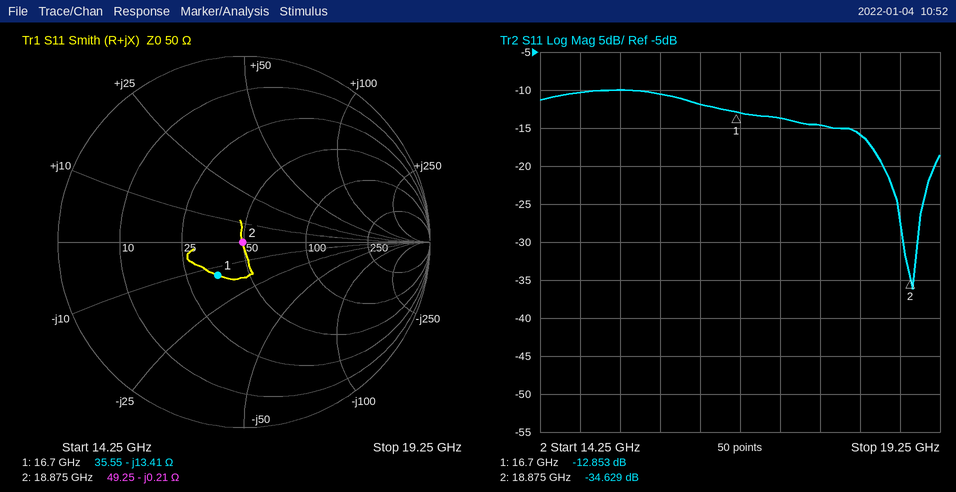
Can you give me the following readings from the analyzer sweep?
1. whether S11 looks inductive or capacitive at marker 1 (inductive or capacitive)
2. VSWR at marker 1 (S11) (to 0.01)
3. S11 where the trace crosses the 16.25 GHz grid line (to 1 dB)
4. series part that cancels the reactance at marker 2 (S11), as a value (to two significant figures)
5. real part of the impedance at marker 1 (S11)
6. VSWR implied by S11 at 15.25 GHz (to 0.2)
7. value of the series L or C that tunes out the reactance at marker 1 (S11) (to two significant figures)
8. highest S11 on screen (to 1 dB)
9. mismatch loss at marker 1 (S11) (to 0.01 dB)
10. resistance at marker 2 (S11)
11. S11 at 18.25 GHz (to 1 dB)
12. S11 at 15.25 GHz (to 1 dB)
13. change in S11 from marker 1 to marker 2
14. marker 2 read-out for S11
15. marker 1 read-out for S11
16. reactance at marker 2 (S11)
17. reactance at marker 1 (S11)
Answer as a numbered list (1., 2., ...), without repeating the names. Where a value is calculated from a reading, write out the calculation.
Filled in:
1. capacitive
2. 1.59
3. -12 dB
4. L = 0.21 Ω/(2π × 18.875 GHz) ≈ 1.8 pH
5. 35.55 Ω
6. |Γ| = 10^(-10/20) = 0.3162; VSWR = (1 + 0.3162)/(1 − 0.3162) ≈ 1.92, so 2.0 to the nearest 0.2
7. L = 13.41 Ω/(2π × 16.7 GHz) ≈ 128 pH, so 130 pH to two significant figures
8. -10 dB
9. −10 log10(1 − 10^(-12.853/10)) ≈ 0.23 dB
10. 49.25 Ω
11. -16 dB
12. -10 dB
13. -34.629 − (-12.853) = -21.776 dB
14. -34.629 dB
15. -12.853 dB
16. -0.21 Ω
17. -13.41 Ω
